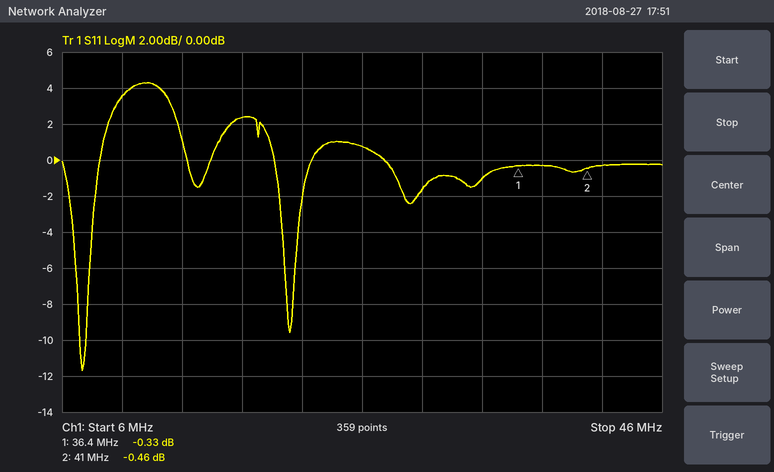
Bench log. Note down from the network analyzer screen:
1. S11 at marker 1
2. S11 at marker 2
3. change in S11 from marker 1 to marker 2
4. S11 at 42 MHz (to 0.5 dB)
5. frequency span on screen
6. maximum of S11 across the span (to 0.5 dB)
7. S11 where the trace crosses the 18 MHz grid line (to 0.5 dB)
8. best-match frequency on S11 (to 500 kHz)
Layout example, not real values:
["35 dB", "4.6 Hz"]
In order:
["-0.33 dB", "-0.46 dB", "-0.13 dB", "-0.5 dB", "40 MHz", "4.5 dB", "2.5 dB", "7.5 MHz"]
